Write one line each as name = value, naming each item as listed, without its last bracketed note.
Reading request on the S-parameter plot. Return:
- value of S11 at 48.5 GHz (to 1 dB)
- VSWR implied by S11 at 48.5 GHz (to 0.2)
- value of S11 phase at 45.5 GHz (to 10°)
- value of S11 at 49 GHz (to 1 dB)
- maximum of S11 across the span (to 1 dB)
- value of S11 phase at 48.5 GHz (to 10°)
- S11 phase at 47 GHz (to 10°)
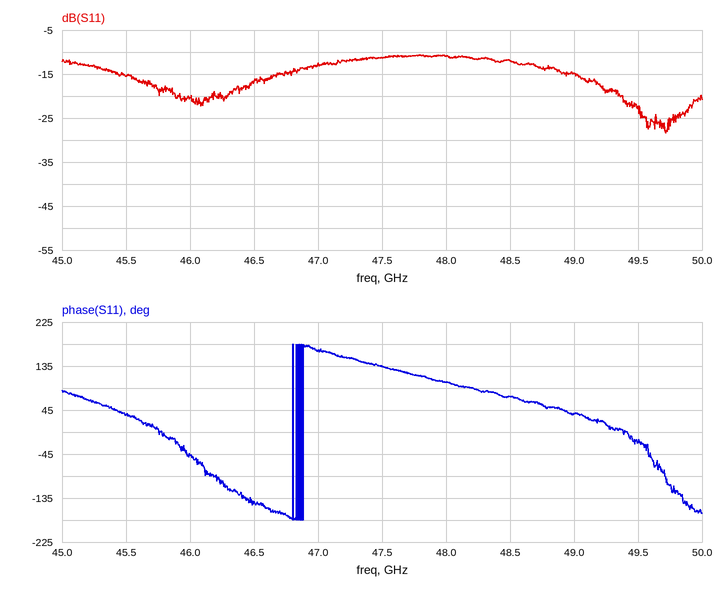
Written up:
value of S11 at 48.5 GHz = -12 dB
VSWR implied by S11 at 48.5 GHz = 1.6
value of S11 phase at 45.5 GHz = 40°
value of S11 at 49 GHz = -15 dB
maximum of S11 across the span = -11 dB
value of S11 phase at 48.5 GHz = 70°
S11 phase at 47 GHz = 170°
